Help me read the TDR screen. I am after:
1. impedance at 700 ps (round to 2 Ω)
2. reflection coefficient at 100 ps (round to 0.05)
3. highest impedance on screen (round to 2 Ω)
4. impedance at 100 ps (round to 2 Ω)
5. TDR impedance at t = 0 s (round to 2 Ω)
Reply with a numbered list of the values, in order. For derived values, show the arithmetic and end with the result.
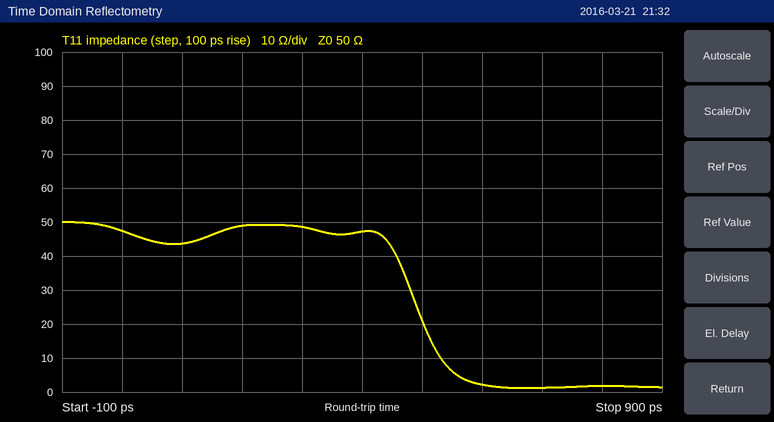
1. 2 Ω
2. (44 − 50)/(44 + 50) ≈ -0.0638, so -0.05 to the nearest 0.05
3. 50 Ω
4. 44 Ω
5. 48 Ω
